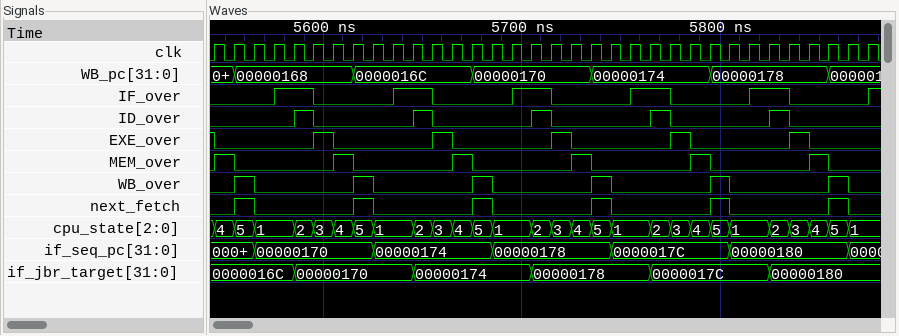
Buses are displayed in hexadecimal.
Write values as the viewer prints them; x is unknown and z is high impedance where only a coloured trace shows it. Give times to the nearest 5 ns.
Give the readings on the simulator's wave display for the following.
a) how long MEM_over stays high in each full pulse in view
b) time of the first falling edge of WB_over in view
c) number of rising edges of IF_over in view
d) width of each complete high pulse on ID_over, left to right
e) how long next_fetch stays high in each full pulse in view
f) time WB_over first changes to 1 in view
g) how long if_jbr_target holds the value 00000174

10 ns, 10 ns, 10 ns, 10 ns, 10 ns, 10 ns
5565 ns
6
10 ns, 10 ns, 10 ns, 10 ns, 10 ns
10 ns, 10 ns, 10 ns, 10 ns, 10 ns, 10 ns
5555 ns
60 ns
